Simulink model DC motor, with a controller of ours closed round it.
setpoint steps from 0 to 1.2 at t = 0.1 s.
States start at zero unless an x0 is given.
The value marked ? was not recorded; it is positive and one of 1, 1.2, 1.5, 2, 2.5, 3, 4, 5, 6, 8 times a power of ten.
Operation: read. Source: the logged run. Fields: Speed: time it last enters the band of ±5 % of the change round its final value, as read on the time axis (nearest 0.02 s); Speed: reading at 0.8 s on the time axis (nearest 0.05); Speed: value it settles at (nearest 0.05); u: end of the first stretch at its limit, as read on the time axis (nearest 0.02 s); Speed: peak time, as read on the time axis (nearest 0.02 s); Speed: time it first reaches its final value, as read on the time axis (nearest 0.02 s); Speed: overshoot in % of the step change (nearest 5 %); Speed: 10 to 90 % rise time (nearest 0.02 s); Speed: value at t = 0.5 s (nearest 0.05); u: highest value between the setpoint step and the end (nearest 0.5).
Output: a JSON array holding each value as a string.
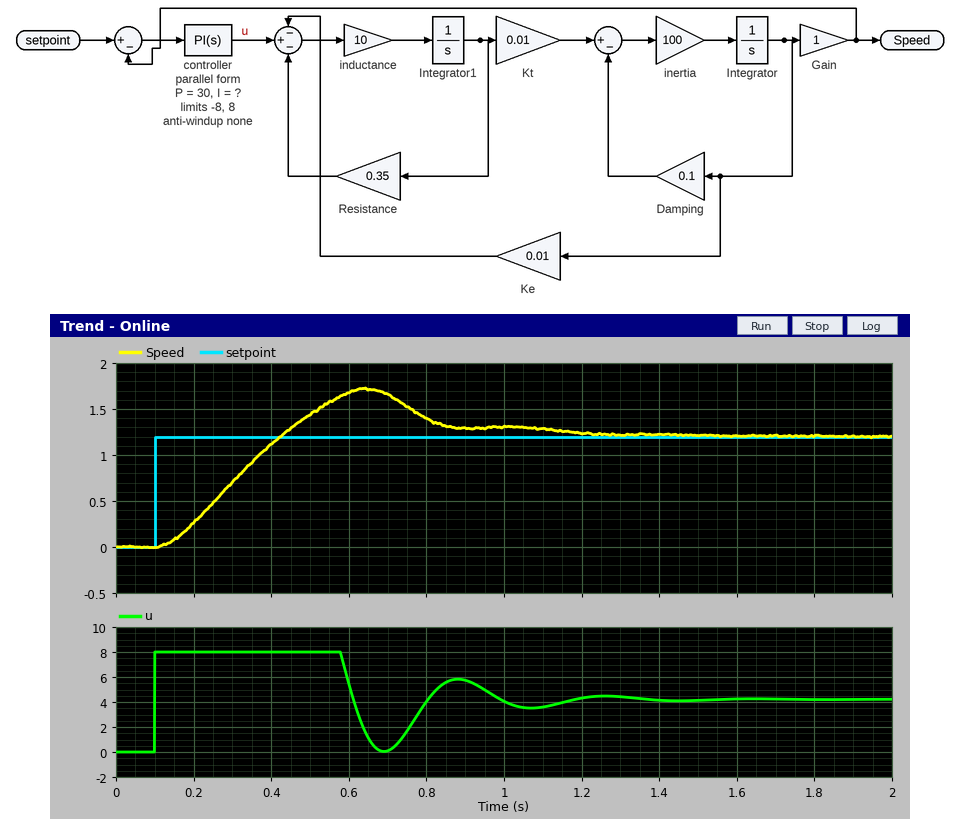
["1.14 s", "1.40", "1.20", "0.58 s", "0.64 s", "0.42 s", "45 %", "0.22 s", "1.45", "8.0"]
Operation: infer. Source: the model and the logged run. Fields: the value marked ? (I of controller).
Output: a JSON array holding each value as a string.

["120"]
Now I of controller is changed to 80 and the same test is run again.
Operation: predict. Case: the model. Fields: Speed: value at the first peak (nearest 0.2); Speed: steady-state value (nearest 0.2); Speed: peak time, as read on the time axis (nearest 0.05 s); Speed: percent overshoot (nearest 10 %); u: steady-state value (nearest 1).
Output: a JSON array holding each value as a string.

["1.6", "1.2", "0.60 s", "30 %", "4"]
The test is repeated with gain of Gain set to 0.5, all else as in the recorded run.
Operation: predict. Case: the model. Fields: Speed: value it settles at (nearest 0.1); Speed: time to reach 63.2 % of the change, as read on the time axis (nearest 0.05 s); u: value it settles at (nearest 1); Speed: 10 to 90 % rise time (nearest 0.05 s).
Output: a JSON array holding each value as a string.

["1.1", "0.50 s", "8", "0.70 s"]
